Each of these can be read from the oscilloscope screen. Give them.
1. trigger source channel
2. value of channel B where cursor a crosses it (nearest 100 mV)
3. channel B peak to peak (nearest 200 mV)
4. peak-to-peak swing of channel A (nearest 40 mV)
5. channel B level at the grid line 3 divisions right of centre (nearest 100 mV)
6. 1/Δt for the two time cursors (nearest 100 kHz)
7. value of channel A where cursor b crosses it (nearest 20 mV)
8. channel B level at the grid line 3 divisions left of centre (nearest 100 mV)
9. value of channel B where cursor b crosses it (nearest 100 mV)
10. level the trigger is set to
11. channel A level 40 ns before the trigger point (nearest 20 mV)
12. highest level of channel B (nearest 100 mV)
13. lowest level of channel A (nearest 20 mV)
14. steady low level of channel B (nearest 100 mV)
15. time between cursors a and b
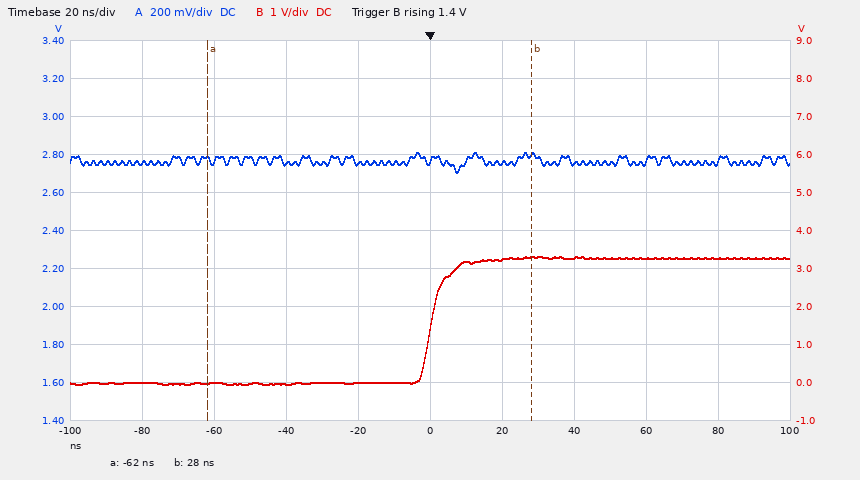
channel B
0.0 V
3.4 V
120 mV
3.3 V
11.1 MHz
2.80 V
0.0 V
3.3 V
1.4 V
2.76 V
3.3 V
2.70 V
0.0 V
90 ns
